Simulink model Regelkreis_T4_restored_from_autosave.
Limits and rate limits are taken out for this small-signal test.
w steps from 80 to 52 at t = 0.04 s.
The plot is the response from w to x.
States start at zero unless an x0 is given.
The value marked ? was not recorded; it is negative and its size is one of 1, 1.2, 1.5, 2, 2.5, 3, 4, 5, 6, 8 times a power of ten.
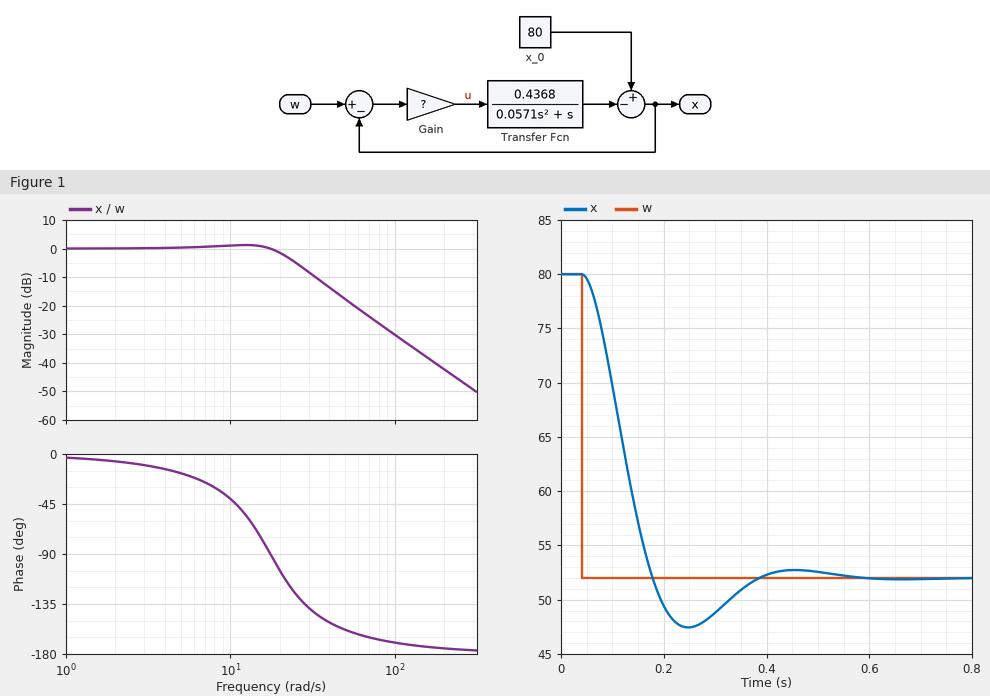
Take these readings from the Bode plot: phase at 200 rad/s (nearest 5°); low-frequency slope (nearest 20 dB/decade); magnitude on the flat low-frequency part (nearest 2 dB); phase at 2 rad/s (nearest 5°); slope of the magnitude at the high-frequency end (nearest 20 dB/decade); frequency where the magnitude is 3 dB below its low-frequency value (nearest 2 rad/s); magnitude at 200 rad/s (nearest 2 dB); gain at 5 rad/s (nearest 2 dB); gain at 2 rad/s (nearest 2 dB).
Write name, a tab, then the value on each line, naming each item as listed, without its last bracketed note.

phase at 200 rad/s	-175°
low-frequency slope	0 dB/decade
magnitude on the flat low-frequency part	0 dB
phase at 2 rad/s	-5°
slope of the magnitude at the high-frequency end	-40 dB/decade
frequency where the magnitude is 3 dB below its low-frequency value	22 rad/s
magnitude at 200 rad/s	-42 dB
gain at 5 rad/s	0 dB
gain at 2 rad/s	0 dB
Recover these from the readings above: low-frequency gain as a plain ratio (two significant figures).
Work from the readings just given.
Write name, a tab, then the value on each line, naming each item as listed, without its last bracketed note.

low-frequency gain as a plain ratio	1.0
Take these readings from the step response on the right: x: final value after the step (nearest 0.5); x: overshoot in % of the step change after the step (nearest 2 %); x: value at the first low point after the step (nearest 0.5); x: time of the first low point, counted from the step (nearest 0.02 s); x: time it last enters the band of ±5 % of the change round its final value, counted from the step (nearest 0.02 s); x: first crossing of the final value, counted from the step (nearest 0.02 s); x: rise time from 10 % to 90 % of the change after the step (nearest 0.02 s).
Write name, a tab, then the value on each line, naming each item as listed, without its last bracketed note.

x: final value after the step	52.0
x: overshoot in % of the step change after the step	16 %
x: value at the first low point after the step	47.5
x: time of the first low point, counted from the step	0.20 s
x: time it last enters the band of ±5 % of the change round its final value, counted from the step	0.30 s
x: first crossing of the final value, counted from the step	0.14 s
x: rise time from 10 % to 90 % of the change after the step	0.10 s
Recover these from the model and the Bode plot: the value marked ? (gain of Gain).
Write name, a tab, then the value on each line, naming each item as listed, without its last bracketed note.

the value marked ?	-40
